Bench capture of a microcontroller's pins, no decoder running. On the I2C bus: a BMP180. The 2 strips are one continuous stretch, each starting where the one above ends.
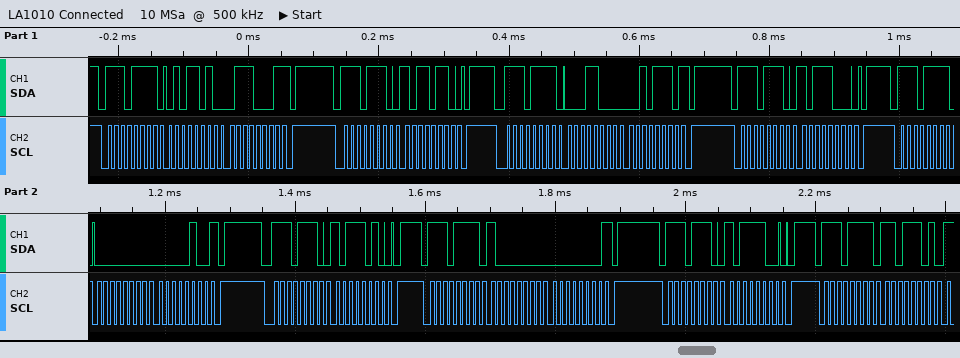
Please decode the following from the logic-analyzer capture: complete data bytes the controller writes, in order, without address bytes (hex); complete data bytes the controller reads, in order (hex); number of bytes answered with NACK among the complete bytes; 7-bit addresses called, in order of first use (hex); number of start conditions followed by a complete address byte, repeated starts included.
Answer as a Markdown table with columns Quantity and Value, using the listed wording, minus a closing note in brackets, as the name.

| Quantity | Value |
|---|---|
| complete data bytes the controller writes, in order, without address bytes | B6 B8 BA BC |
| complete data bytes the controller reads, in order | 5A 71 18 2E 00 04 80 00 DD |
| number of bytes answered with NACK among the complete bytes | 4 |
| 7-bit addresses called, in order of first use | 0x77 |
| number of start conditions followed by a complete address byte, repeated starts included | 9 |
